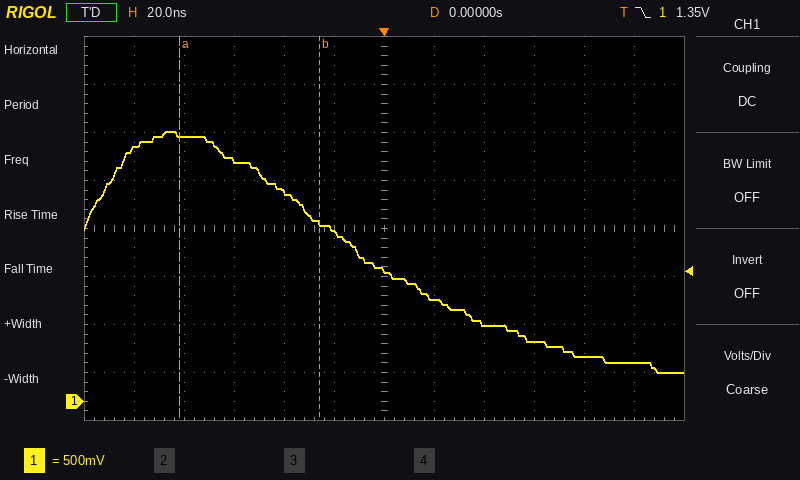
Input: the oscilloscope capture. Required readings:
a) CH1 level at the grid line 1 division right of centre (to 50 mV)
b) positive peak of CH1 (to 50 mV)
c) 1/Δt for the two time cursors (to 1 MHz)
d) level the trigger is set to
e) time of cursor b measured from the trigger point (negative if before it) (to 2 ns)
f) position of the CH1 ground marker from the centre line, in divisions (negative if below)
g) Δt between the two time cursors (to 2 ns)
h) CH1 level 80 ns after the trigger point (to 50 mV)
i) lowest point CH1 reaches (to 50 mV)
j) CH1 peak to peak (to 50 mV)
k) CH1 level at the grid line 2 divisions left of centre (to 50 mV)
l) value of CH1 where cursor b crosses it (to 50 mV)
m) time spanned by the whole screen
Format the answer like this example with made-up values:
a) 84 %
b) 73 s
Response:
a) 1.05 V
b) 2.80 V
c) 18 MHz
d) 1.35 V
e) -26 ns
f) -3.6 div
g) 56 ns
h) 450 mV
i) 300 mV
j) 2.50 V
k) 2.20 V
l) 1.85 V
m) 240 ns
